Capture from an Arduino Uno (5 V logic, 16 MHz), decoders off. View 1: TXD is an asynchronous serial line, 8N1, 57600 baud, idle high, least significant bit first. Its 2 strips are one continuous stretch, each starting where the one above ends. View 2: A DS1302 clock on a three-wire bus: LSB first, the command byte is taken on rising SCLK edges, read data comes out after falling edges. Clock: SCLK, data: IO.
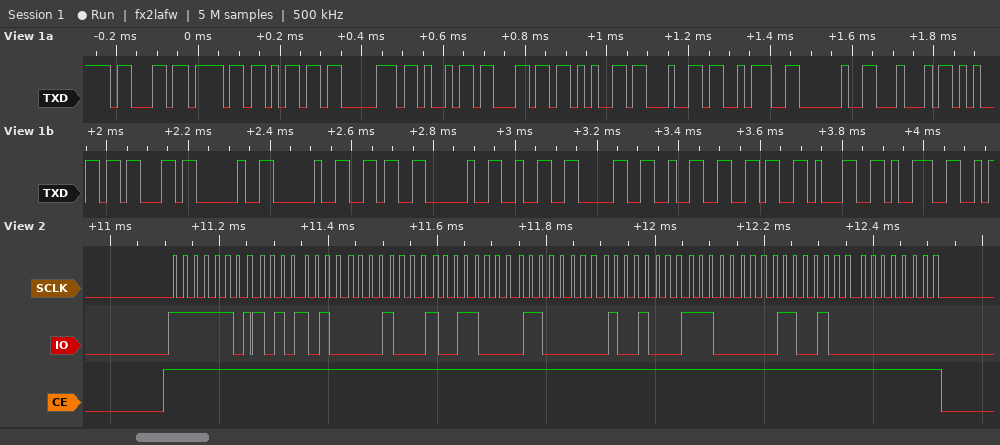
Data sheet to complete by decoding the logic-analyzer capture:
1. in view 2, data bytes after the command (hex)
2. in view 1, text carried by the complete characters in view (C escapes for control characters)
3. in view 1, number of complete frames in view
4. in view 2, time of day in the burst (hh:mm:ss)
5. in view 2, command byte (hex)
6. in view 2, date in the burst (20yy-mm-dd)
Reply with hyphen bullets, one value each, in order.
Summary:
- 55 10 19 06 12 07 26 00
- "compiled: Dec  6 202619"
- 23
- 19:10:55
- 0xBF
- 2026-12-06
